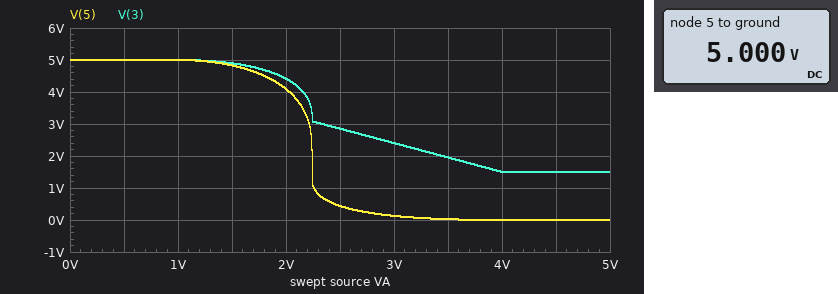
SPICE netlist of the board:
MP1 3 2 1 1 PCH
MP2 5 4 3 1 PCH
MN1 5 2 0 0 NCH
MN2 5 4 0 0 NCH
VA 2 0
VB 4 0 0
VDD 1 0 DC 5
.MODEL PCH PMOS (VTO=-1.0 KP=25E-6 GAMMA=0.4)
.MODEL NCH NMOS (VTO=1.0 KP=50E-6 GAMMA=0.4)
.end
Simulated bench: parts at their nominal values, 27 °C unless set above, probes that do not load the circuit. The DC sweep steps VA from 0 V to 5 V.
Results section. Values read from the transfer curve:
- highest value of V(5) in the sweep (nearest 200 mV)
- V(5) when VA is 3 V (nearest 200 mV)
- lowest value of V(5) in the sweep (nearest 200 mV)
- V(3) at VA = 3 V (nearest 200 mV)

5.0 V
200 mV
0 V
2.4 V
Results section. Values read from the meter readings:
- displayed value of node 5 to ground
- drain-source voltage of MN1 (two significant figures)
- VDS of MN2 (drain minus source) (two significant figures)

5.000 V
5.0 V
5.0 V
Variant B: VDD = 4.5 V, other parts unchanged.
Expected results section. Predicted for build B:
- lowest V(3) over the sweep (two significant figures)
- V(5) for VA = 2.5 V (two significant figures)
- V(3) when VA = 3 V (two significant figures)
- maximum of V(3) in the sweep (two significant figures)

1.5 V
180 mV
1.9 V
4.5 V
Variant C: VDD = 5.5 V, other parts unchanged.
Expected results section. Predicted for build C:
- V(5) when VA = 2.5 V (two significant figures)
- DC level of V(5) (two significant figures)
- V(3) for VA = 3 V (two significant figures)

1.0 V
5.5 V
2.9 V
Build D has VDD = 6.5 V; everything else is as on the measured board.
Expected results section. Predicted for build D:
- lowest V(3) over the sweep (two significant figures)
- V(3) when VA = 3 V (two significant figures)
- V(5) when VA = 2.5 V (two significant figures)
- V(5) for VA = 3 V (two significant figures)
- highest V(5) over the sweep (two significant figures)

2.1 V
3.9 V
5.1 V
1.1 V
6.5 V
